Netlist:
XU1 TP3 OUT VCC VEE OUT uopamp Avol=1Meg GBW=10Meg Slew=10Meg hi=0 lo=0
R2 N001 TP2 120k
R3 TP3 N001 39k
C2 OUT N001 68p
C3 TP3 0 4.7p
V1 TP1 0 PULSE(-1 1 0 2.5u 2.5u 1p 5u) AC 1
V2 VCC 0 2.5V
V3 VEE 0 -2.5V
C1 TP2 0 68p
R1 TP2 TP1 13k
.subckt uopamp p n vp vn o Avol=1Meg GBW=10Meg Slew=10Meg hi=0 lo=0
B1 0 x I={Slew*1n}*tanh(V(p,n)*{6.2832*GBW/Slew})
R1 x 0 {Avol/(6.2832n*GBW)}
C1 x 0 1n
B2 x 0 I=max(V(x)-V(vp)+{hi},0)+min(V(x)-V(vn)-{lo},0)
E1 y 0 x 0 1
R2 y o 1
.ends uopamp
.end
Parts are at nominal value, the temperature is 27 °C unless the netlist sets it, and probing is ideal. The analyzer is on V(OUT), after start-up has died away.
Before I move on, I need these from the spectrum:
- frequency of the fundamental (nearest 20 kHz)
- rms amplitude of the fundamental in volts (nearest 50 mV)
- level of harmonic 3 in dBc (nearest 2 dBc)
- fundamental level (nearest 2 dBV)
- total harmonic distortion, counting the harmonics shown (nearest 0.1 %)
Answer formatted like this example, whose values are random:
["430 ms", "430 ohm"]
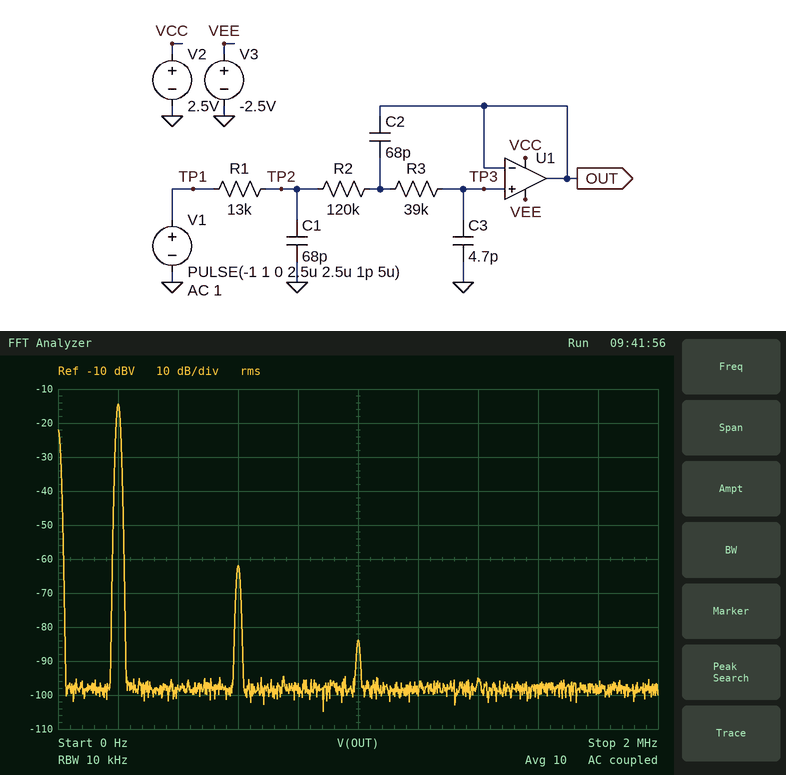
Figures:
["200 kHz", "200 mV", "-48 dBc", "-14 dBV", "0.4 %"]
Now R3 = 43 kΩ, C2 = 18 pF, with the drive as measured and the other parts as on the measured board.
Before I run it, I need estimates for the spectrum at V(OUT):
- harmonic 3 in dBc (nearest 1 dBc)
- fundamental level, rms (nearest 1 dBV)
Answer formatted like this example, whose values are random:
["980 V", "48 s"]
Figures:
["-42 dBc", "-9 dBV"]
